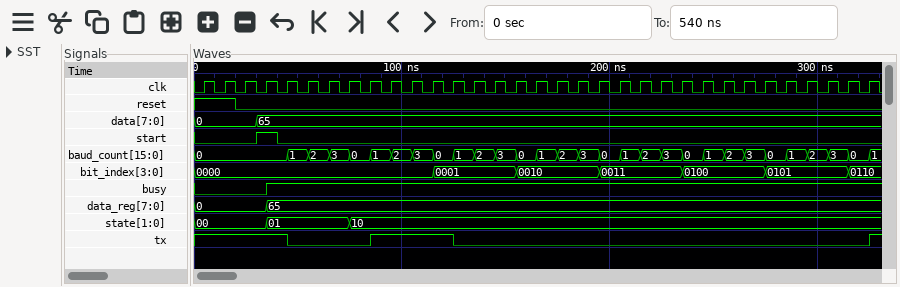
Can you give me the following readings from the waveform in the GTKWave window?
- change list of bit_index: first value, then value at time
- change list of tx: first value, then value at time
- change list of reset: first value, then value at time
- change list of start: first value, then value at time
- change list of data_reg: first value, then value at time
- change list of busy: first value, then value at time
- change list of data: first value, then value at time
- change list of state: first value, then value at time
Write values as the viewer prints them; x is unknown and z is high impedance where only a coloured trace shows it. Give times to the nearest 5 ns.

0000, 0001 at 115 ns, 0010 at 155 ns, 0011 at 195 ns, 0100 at 235 ns, 0101 at 275 ns, 0110 at 315 ns
1, 0 at 45 ns, 1 at 85 ns, 0 at 125 ns, 1 at 325 ns
1, 0 at 20 ns
0, 1 at 30 ns, 0 at 40 ns
0, 65 at 35 ns
0, 1 at 35 ns
0, 65 at 30 ns
00, 01 at 35 ns, 10 at 75 ns
